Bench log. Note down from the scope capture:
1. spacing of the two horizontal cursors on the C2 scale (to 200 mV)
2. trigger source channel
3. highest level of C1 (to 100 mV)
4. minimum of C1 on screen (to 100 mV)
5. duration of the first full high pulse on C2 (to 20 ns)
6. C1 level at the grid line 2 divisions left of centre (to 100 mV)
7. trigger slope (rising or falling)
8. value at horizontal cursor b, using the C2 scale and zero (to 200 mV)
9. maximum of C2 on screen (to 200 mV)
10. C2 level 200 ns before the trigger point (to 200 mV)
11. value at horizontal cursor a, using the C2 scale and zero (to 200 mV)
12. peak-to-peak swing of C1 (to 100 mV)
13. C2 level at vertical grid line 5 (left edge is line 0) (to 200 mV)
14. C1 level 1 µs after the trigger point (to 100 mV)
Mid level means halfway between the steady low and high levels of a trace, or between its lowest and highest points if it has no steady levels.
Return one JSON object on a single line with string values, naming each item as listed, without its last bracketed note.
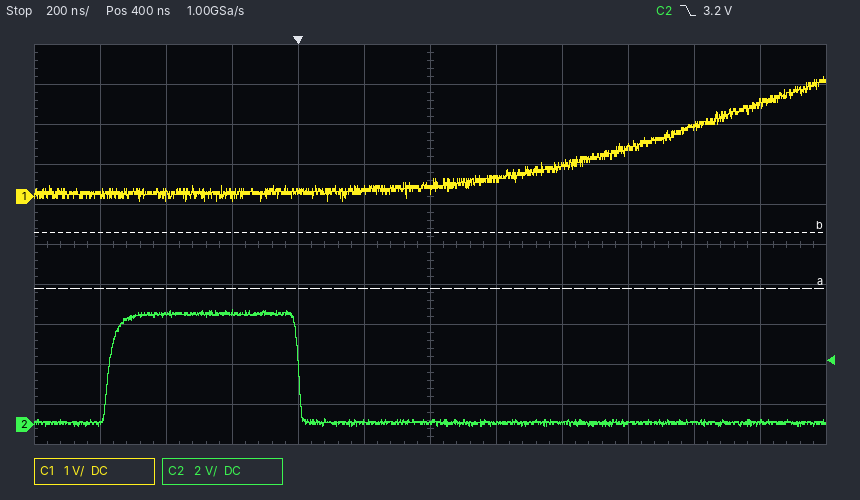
{"spacing of the two horizontal cursors on the C2 scale": "2.8 V", "trigger source channel": "C2", "highest level of C1": "3.0 V", "minimum of C1 on screen": "-100 mV", "duration of the first full high pulse on C2": "580 ns", "C1 level at the grid line 2 divisions left of centre": "100 mV", "trigger slope": "falling", "value at horizontal cursor b, using the C2 scale and zero": "9.6 V", "maximum of C2 on screen": "5.8 V", "C2 level 200 ns before the trigger point": "5.6 V", "value at horizontal cursor a, using the C2 scale and zero": "6.8 V", "peak-to-peak swing of C1": "3.1 V", "C2 level at vertical grid line 5 (left edge is line 0)": "200 mV", "C1 level 1 µs after the trigger point": "1.2 V"}
